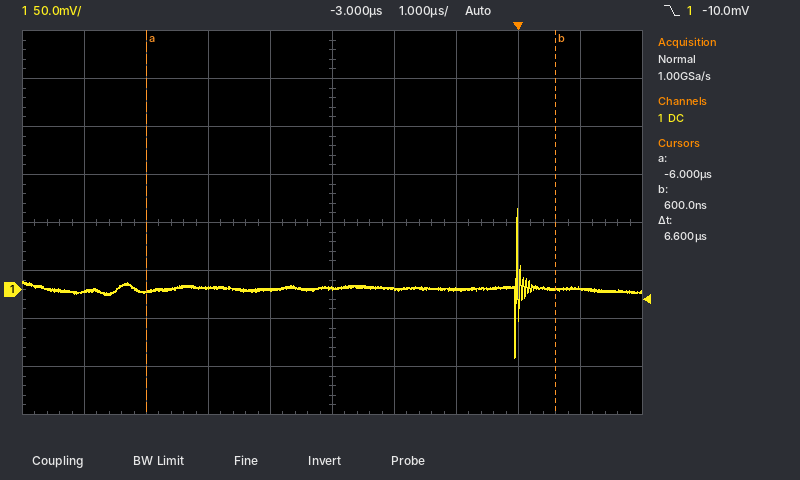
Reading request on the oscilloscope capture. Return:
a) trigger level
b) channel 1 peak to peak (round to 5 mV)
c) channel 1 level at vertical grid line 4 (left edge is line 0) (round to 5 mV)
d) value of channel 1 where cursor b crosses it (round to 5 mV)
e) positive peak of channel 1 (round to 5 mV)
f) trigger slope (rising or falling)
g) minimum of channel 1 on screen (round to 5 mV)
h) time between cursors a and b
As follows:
-10.0 mV
155 mV
0 mV
0 mV
85 mV
falling
-70 mV
6.6 µs
